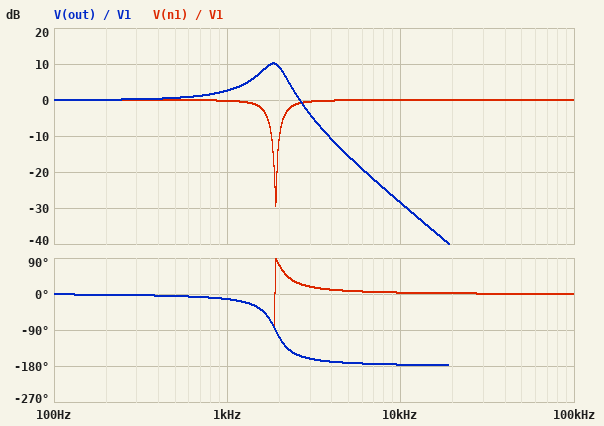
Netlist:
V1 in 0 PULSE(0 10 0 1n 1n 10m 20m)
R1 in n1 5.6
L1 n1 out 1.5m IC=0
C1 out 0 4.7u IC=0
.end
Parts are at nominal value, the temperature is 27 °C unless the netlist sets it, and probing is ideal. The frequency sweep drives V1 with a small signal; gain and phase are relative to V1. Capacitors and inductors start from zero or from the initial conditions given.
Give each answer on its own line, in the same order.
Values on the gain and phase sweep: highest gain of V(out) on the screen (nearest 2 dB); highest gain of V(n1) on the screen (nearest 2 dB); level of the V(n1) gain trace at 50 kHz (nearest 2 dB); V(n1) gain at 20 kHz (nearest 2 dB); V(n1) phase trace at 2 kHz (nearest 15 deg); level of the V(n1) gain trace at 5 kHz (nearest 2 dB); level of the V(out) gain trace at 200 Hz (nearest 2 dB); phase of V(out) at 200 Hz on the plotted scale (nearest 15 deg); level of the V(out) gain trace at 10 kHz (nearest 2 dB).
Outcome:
10 dB
0 dB
0 dB
0 dB
75 deg
0 dB
0 dB
0 deg
-28 dB
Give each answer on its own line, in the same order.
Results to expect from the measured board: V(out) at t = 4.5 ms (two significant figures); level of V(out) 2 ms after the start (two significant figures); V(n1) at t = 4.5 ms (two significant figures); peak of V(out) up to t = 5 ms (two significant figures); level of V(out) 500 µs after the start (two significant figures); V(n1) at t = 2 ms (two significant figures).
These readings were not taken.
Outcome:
10 V
10 V
10 V
16 V
6.6 V
10 V
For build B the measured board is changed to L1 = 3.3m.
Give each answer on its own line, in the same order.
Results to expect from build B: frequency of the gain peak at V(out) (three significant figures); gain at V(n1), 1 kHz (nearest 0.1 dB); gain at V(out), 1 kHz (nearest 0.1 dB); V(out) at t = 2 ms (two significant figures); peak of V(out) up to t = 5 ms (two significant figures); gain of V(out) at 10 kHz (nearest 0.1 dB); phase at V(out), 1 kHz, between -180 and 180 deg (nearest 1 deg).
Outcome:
1.26 kHz
-0.7 dB
7.5 dB
12 V
17 V
-35.6 dB
-23 deg
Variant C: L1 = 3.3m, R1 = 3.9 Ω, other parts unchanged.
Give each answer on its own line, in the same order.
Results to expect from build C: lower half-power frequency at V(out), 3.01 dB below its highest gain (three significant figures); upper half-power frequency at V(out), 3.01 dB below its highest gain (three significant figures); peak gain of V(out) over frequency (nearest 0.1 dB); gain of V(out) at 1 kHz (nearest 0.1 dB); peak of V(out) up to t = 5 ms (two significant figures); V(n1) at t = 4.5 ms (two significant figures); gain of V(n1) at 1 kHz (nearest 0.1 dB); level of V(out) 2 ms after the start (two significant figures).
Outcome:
1.17 kHz
1.36 kHz
16.7 dB
7.9 dB
18 V
10 V
-0.4 dB
13 V
